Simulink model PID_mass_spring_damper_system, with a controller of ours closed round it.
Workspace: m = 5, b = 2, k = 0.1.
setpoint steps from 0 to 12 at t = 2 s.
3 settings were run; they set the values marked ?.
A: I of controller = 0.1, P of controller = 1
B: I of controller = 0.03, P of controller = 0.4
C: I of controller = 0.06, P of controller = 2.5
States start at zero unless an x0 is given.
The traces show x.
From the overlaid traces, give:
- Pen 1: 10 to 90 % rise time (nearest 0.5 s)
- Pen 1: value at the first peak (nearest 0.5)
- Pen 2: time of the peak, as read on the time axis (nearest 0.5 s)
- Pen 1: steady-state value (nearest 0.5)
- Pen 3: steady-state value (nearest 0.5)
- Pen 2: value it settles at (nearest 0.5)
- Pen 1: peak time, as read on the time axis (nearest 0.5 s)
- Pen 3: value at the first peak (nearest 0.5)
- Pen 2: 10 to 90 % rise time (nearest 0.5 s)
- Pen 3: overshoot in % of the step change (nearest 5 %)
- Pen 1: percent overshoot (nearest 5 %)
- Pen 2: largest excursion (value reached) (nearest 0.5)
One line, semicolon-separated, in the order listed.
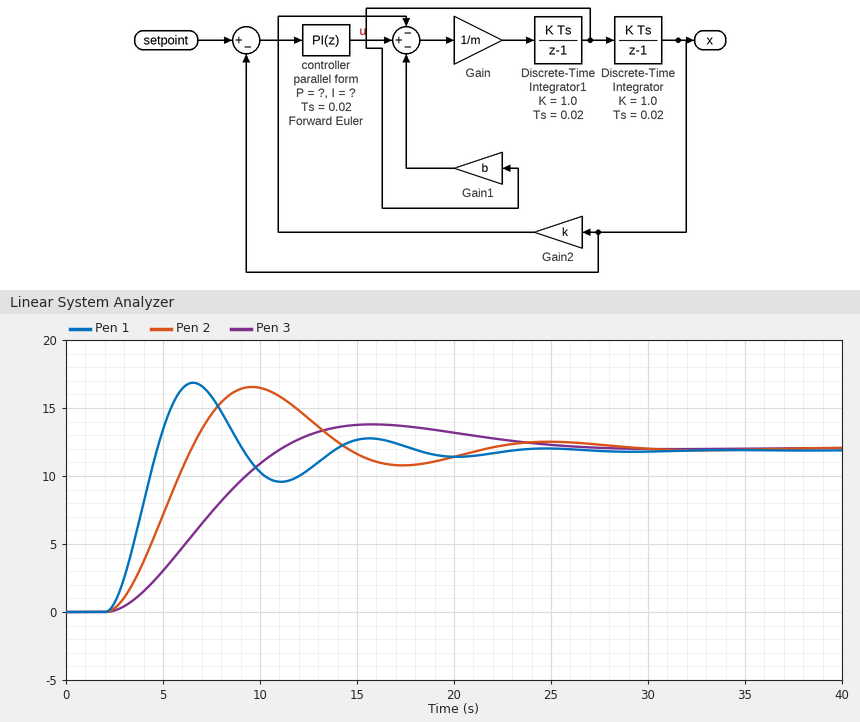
2.0 s; 17.0; 9.5 s; 12.0; 12.0; 12.0; 6.5 s; 14.0; 3.0 s; 15 %; 40 %; 16.5
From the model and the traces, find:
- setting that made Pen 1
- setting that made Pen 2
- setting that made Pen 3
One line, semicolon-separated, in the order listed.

C; A; B
